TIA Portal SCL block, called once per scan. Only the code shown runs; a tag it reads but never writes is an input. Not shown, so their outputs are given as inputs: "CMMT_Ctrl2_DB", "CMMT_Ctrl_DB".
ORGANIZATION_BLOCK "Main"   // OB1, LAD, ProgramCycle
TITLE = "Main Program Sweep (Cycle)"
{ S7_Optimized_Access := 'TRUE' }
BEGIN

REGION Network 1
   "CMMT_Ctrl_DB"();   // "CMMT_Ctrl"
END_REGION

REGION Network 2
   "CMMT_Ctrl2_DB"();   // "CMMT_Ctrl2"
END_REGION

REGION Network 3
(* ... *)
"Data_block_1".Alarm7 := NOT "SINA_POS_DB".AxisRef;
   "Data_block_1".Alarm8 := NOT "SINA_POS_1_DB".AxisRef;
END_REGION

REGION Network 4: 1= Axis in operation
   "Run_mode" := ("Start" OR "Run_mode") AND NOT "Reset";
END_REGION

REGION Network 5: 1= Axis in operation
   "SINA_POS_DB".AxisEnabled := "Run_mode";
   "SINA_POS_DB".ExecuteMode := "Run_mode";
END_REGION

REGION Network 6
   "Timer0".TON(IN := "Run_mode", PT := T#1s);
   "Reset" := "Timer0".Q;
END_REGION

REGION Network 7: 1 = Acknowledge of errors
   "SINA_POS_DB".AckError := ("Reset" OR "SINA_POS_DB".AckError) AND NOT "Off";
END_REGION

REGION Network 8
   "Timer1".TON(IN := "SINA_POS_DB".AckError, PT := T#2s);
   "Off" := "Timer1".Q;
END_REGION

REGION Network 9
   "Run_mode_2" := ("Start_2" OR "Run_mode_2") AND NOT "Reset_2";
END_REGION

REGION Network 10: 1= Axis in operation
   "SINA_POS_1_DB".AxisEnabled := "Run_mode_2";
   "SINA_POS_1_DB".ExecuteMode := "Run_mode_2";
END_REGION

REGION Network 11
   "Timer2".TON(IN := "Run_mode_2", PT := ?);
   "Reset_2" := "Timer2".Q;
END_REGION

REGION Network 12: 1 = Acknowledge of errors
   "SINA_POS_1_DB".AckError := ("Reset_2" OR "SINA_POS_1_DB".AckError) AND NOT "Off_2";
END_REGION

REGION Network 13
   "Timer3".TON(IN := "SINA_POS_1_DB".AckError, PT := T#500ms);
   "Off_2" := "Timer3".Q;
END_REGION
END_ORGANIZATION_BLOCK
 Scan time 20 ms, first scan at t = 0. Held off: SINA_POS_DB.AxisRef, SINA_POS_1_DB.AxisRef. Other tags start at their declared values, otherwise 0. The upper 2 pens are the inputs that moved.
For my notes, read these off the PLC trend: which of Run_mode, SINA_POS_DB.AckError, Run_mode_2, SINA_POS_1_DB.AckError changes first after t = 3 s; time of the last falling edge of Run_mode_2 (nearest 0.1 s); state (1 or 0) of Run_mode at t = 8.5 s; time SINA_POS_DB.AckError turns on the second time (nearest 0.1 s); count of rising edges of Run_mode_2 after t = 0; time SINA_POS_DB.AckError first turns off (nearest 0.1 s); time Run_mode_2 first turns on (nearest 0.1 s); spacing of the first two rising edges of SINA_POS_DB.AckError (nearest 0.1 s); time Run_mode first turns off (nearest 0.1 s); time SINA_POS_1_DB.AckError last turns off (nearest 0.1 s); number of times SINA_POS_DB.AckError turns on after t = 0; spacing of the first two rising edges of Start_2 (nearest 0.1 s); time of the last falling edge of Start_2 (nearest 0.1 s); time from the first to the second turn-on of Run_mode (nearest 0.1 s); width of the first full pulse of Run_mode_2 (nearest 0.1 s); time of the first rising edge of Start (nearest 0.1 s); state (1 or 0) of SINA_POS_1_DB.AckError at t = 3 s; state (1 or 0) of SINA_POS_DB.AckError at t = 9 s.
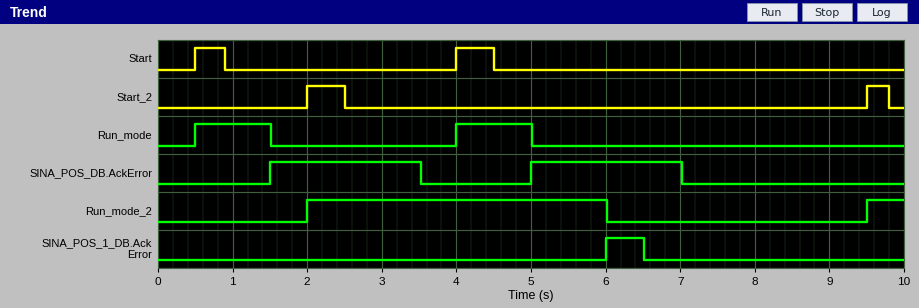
SINA_POS_DB.AckError
6.0 s
0
5.0 s
2
3.5 s
2.0 s
3.5 s
1.5 s
6.5 s
2
7.5 s
9.8 s
3.5 s
4.0 s
0.5 s
0
0
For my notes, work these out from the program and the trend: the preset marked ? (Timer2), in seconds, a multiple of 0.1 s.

4.0 s
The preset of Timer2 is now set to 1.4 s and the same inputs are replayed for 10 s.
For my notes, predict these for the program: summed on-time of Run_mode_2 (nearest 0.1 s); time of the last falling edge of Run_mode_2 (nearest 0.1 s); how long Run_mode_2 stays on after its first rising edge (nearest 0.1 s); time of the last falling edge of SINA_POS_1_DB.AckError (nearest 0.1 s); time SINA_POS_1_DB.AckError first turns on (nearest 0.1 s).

1.9 s
3.4 s
1.4 s
3.9 s
3.4 s
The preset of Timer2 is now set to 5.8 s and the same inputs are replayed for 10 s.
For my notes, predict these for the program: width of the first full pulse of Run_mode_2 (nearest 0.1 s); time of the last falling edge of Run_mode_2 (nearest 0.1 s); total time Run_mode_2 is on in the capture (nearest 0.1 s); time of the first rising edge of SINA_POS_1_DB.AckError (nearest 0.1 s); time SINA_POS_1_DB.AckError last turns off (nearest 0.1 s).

5.8 s
7.8 s
6.3 s
7.8 s
8.3 s
